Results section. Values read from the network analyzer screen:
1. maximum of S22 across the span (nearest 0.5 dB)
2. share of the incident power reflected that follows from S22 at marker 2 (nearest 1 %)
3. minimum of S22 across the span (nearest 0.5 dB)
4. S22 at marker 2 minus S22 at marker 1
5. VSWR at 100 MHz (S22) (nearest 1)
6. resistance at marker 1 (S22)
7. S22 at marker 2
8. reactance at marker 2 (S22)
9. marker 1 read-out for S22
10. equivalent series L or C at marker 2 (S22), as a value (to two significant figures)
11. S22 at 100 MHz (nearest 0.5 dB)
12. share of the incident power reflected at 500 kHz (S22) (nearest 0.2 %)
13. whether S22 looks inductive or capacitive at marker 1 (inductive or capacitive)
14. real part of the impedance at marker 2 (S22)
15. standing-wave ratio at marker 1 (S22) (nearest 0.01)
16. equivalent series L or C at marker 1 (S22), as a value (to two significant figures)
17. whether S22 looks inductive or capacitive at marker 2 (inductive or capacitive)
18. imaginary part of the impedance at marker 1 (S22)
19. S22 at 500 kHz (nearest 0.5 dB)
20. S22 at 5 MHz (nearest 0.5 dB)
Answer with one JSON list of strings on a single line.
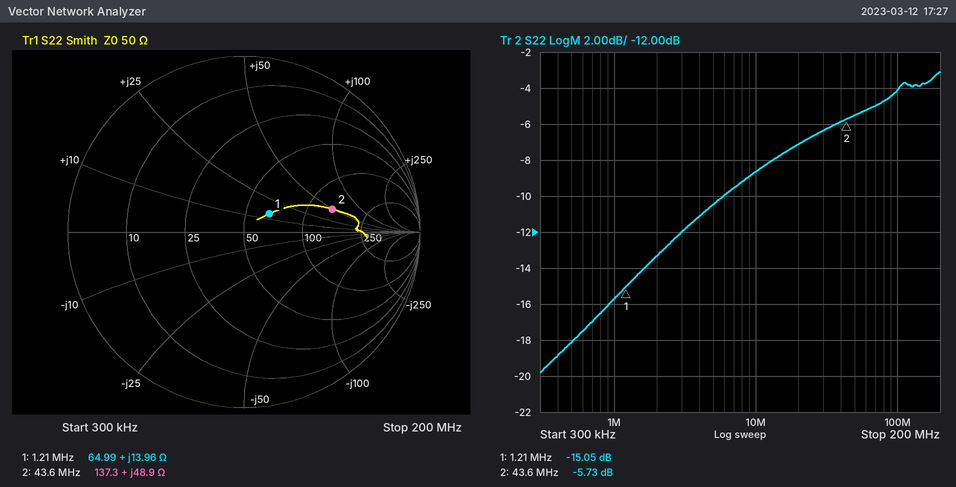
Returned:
["-3.0 dB", "27 %", "-20.0 dB", "9.32 dB", "4", "64.99 Ω", "-5.73 dB", "+48.9 Ω", "-15.05 dB", "180 nH", "-4.0 dB", "1.6 %", "inductive", "137.3 Ω", "1.43", "1.8 µH", "inductive", "+13.96 Ω", "-18.0 dB", "-10.5 dB"]
